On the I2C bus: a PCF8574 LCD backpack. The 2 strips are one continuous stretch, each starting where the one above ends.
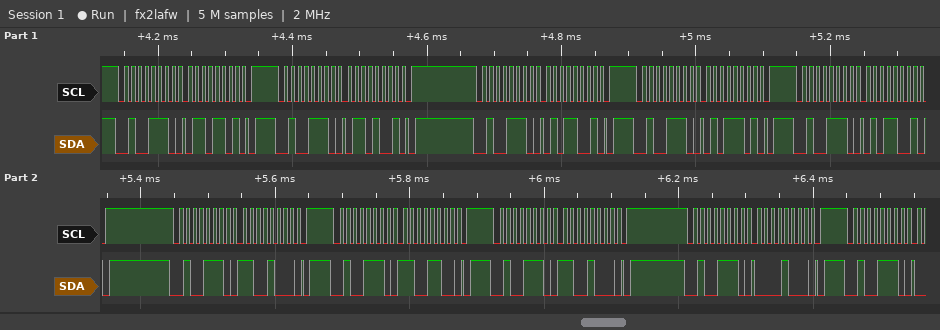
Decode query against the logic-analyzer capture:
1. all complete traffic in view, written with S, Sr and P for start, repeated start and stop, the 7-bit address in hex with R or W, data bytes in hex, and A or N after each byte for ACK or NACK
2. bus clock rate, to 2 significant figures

S 27W A 6D A P S 27W A 69 A P S 27W A 59 A P S 27W A 5D A P S 27W A 59 A P S 27W A C8 A P S 27W A CC A P S 27W A C8 A P S 27W A 08 A P S 27W A
100 kHz
